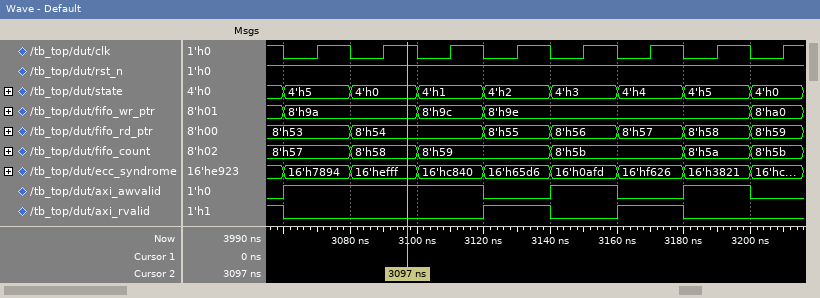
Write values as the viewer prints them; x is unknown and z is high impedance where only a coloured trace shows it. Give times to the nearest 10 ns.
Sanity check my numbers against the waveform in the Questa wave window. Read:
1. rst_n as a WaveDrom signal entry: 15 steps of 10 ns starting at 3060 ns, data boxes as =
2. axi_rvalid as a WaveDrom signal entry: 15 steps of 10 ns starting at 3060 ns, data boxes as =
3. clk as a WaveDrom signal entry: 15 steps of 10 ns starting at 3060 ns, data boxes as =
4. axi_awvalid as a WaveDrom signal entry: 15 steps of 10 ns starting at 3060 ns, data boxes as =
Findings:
{name: 'rst_n', wave: '1..............'}
{name: 'axi_rvalid', wave: '0.....1.0.1.0..'}
{name: 'clk', wave: '010101010101010'}
{name: 'axi_awvalid', wave: '1.....0.1.0.1.0'}
